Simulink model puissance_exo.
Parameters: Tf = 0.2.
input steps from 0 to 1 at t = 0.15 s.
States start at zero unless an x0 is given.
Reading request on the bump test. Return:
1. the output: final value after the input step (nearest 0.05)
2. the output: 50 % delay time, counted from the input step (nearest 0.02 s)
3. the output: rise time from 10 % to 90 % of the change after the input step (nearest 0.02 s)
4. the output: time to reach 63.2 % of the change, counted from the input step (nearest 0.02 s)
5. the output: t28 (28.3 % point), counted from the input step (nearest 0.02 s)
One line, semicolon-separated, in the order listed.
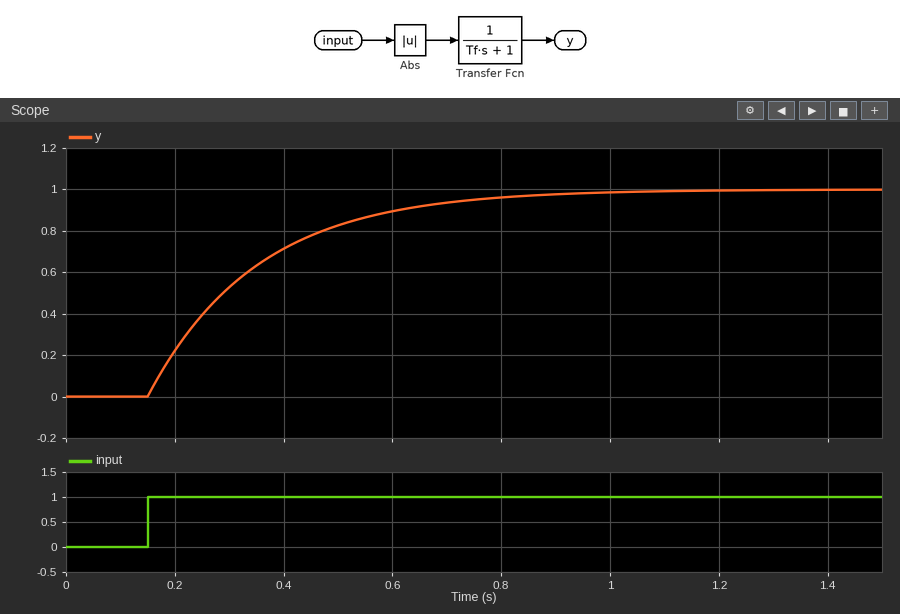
1.00; 0.14 s; 0.44 s; 0.20 s; 0.06 s
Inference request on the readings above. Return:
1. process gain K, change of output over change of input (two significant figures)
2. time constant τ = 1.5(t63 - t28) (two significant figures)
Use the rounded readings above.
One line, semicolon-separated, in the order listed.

1.0; 0.21 s
